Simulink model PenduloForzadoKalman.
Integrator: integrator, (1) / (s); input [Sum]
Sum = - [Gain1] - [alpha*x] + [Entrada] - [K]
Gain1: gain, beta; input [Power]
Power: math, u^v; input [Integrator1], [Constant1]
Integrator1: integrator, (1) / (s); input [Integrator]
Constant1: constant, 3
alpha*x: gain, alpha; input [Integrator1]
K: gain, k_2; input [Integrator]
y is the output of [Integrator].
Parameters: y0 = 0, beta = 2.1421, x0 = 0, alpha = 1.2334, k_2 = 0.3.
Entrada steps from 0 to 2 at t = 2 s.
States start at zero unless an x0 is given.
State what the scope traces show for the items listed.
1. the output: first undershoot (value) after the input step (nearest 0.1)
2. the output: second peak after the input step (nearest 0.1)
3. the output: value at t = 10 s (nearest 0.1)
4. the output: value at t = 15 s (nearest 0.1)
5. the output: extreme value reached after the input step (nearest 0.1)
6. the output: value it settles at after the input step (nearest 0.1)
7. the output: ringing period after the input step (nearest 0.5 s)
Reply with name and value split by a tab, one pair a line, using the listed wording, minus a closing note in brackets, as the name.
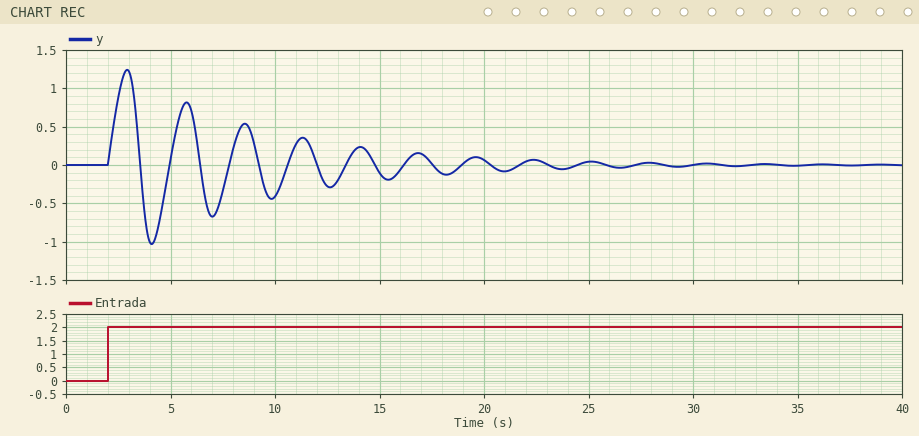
the output: first undershoot (value) after the input step	-1.0
the output: second peak after the input step	0.8
the output: value at t = 10 s	-0.4
the output: value at t = 15 s	-0.1
the output: extreme value reached after the input step	1.2
the output: value it settles at after the input step	0.0
the output: ringing period after the input step	3.0 s
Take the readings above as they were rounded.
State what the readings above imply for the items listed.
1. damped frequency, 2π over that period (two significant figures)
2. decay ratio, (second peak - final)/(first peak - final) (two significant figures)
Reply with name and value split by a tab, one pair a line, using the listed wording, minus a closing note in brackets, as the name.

damped frequency, 2π over that period	2.1 rad/s
decay ratio, (second peak - final)/(first peak - final)	0.67
